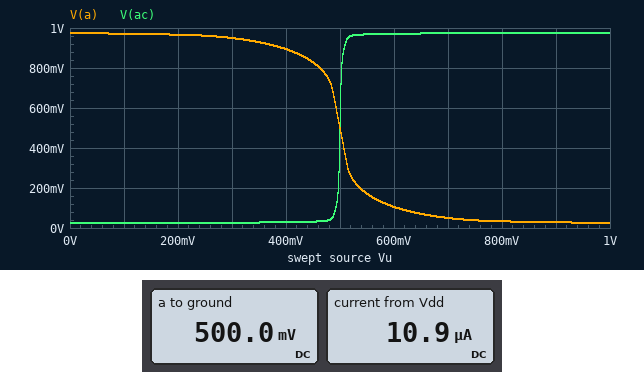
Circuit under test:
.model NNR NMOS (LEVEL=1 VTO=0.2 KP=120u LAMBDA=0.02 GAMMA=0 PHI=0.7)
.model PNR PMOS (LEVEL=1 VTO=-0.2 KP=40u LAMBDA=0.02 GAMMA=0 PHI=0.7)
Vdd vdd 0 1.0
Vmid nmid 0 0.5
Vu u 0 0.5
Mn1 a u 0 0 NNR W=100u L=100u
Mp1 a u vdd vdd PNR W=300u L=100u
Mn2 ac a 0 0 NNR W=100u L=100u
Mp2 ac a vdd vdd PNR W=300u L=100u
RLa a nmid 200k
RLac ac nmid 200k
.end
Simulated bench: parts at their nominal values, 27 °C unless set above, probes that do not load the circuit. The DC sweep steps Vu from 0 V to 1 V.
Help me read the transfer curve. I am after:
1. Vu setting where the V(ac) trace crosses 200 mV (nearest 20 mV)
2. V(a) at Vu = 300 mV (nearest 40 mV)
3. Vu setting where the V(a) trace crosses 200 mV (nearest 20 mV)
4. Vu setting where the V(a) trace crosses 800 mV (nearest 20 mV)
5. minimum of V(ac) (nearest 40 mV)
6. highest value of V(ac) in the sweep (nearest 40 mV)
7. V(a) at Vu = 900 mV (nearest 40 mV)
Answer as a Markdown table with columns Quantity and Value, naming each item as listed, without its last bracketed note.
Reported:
| Quantity | Value |
|---|---|
| Vu setting where the V(ac) trace crosses 200 mV | 500 mV |
| V(a) at Vu = 300 mV | 960 mV |
| Vu setting where the V(a) trace crosses 200 mV | 540 mV |
| Vu setting where the V(a) trace crosses 800 mV | 460 mV |
| minimum of V(ac) | 40 mV |
| highest value of V(ac) in the sweep | 960 mV |
| V(a) at Vu = 900 mV | 40 mV |
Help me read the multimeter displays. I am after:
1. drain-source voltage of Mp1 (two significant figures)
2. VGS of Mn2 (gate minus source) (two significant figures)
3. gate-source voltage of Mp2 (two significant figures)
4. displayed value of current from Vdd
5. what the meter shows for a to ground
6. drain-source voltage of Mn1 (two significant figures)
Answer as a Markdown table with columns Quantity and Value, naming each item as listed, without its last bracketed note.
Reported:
| Quantity | Value |
|---|---|
| drain-source voltage of Mp1 | -500 mV |
| VGS of Mn2 (gate minus source) | 500 mV |
| gate-source voltage of Mp2 | -500 mV |
| displayed value of current from Vdd | 10.9 µA |
| what the meter shows for a to ground | 500.0 mV |
| drain-source voltage of Mn1 | 500 mV |
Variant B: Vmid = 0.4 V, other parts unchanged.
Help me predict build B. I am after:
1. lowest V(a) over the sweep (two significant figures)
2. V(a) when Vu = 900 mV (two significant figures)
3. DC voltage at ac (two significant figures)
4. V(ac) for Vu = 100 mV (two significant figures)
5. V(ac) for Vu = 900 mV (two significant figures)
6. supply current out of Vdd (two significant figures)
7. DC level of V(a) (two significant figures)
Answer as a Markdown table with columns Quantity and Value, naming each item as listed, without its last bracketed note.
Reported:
| Quantity | Value |
|---|---|
| lowest V(a) over the sweep | 20 mV |
| V(a) when Vu = 900 mV | 23 mV |
| DC voltage at ac | 880 mV |
| V(ac) for Vu = 100 mV | 21 mV |
| V(ac) for Vu = 900 mV | 970 mV |
| supply current out of Vdd | 10 µA |
| DC level of V(a) | 400 mV |
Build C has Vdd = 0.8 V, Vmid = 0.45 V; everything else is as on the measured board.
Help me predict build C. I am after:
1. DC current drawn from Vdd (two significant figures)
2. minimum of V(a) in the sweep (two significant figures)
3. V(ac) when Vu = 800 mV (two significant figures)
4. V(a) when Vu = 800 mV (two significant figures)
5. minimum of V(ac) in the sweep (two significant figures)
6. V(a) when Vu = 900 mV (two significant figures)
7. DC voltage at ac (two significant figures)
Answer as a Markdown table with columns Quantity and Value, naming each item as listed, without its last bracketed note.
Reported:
| Quantity | Value |
|---|---|
| DC current drawn from Vdd | 2.2 µA |
| minimum of V(a) in the sweep | 23 mV |
| V(ac) when Vu = 800 mV | 780 mV |
| V(a) when Vu = 800 mV | 30 mV |
| minimum of V(ac) in the sweep | 31 mV |
| V(a) when Vu = 900 mV | 26 mV |
| DC voltage at ac | 770 mV |
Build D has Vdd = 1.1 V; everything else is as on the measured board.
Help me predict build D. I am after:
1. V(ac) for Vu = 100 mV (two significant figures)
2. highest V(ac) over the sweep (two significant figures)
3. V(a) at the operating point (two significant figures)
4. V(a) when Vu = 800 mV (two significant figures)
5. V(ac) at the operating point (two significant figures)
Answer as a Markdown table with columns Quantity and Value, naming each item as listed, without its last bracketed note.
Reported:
| Quantity | Value |
|---|---|
| V(ac) for Vu = 100 mV | 23 mV |
| highest V(ac) over the sweep | 1.1 V |
| V(a) at the operating point | 890 mV |
| V(a) when Vu = 800 mV | 42 mV |
| V(ac) at the operating point | 29 mV |
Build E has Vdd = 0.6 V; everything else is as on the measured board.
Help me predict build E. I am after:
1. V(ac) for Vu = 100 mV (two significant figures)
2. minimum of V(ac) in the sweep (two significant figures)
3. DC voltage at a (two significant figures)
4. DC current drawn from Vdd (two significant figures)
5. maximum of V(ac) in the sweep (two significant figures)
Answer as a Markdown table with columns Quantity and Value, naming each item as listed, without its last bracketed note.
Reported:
| Quantity | Value |
|---|---|
| V(ac) for Vu = 100 mV | 52 mV |
| minimum of V(ac) in the sweep | 51 mV |
| DC voltage at a | 68 mV |
| DC current drawn from Vdd | 440 nA |
| maximum of V(ac) in the sweep | 590 mV |
